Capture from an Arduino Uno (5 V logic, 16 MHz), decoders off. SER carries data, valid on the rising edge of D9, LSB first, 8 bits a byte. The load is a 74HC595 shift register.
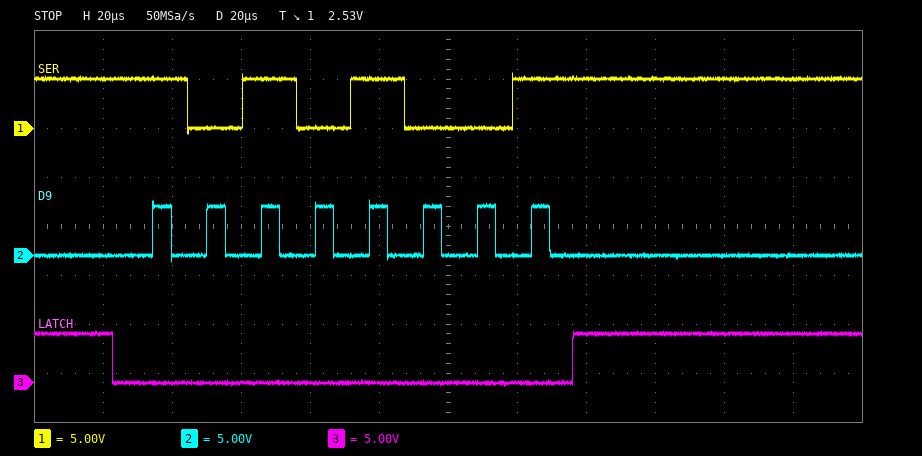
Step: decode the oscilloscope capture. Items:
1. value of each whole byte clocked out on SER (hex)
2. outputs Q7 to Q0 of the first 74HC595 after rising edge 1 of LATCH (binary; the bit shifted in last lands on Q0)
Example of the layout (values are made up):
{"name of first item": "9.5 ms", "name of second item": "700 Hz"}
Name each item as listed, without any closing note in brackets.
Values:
{"value of each whole byte clocked out on SER": "95", "outputs Q7 to Q0 of the first 74HC595 after rising edge 1 of LATCH": "10101001"}
